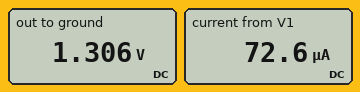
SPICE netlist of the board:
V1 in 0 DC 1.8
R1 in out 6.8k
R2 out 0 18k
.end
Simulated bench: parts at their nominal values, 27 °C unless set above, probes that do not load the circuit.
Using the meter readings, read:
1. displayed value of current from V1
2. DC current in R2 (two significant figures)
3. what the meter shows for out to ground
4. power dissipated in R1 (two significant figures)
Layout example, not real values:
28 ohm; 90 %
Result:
72.6 µA; 73 µA; 1.306 V; 36 µW
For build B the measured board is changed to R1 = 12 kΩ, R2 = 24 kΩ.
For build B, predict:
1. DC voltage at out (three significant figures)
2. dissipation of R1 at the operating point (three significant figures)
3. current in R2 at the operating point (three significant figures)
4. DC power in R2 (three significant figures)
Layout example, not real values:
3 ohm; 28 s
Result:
1.20 V; 30.0 µW; 50.0 µA; 60.0 µW
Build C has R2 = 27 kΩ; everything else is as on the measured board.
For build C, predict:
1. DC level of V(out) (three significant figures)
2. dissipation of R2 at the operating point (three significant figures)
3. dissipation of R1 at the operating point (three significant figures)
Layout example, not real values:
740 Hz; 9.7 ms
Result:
1.44 V; 76.6 µW; 19.3 µW
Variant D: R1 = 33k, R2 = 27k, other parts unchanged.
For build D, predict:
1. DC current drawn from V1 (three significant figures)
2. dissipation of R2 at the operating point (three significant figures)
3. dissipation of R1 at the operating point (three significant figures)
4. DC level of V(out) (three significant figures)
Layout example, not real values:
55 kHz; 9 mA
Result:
30.0 µA; 24.3 µW; 29.7 µW; 810 mV
